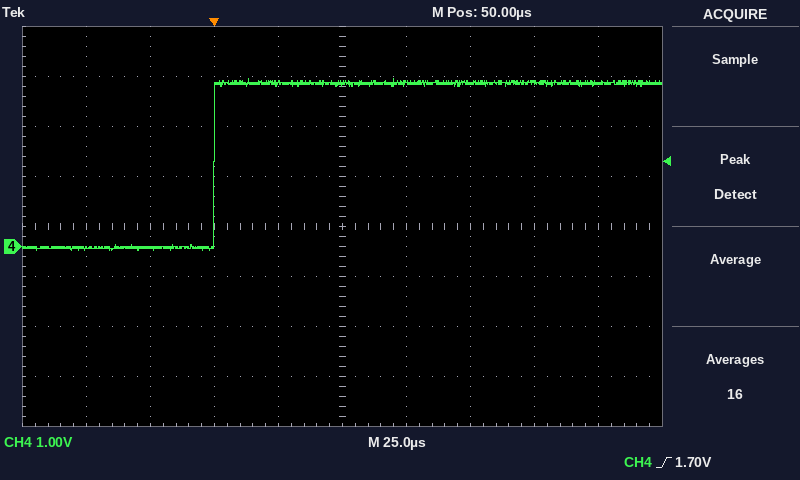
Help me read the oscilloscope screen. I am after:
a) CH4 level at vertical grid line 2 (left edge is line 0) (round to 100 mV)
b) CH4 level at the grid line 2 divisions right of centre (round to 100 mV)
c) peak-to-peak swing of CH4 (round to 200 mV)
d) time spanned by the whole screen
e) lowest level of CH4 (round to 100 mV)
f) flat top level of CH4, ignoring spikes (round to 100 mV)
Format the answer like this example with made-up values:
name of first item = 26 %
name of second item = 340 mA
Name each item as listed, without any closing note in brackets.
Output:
CH4 level at vertical grid line 2 (left edge is line 0) = 0.0 V
CH4 level at the grid line 2 divisions right of centre = 3.3 V
peak-to-peak swing of CH4 = 3.4 V
time spanned by the whole screen = 250 µs
lowest level of CH4 = -100 mV
flat top level of CH4, ignoring spikes = 3.3 V
